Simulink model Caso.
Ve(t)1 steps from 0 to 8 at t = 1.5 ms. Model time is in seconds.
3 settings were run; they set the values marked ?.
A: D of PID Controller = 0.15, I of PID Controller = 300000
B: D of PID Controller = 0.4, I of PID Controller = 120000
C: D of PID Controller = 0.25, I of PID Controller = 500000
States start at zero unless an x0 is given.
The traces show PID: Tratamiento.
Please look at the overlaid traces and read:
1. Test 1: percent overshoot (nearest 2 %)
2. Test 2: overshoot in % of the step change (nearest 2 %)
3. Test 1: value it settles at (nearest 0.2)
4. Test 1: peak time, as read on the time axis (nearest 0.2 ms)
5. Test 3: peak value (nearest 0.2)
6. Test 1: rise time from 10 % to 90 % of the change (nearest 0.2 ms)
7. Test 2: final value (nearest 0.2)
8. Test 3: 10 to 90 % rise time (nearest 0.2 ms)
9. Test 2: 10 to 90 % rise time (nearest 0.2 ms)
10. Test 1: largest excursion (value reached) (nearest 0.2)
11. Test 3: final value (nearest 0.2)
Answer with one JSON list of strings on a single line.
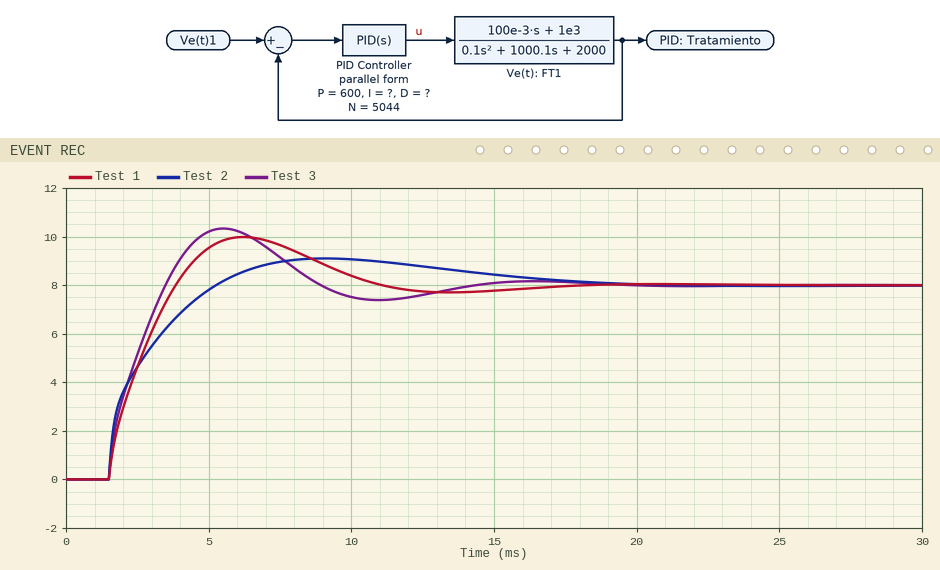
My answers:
["24 %", "14 %", "8.0", "6.2 ms", "10.4", "1.8 ms", "8.0", "1.6 ms", "2.8 ms", "10.0", "8.0"]
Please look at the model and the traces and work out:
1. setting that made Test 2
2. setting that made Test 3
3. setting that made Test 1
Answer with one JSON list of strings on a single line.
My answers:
["B", "C", "A"]
